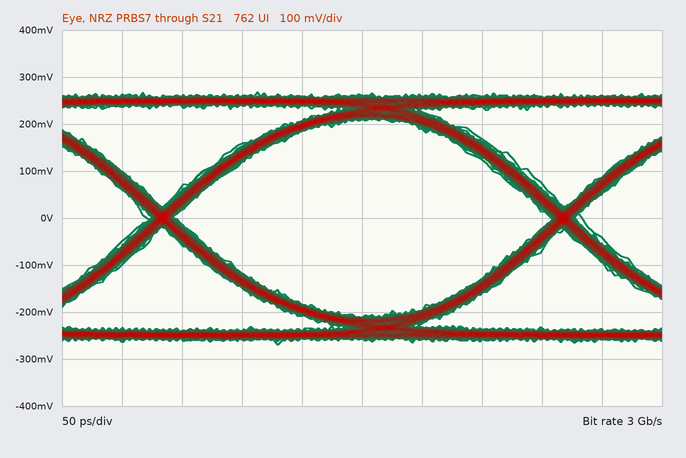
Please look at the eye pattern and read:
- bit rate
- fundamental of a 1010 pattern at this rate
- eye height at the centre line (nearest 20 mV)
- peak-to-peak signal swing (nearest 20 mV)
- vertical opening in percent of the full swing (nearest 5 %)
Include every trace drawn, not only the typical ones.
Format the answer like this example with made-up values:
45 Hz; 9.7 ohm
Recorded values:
3 Gb/s; 1.5 GHz; 420 mV; 540 mV; 80 %
